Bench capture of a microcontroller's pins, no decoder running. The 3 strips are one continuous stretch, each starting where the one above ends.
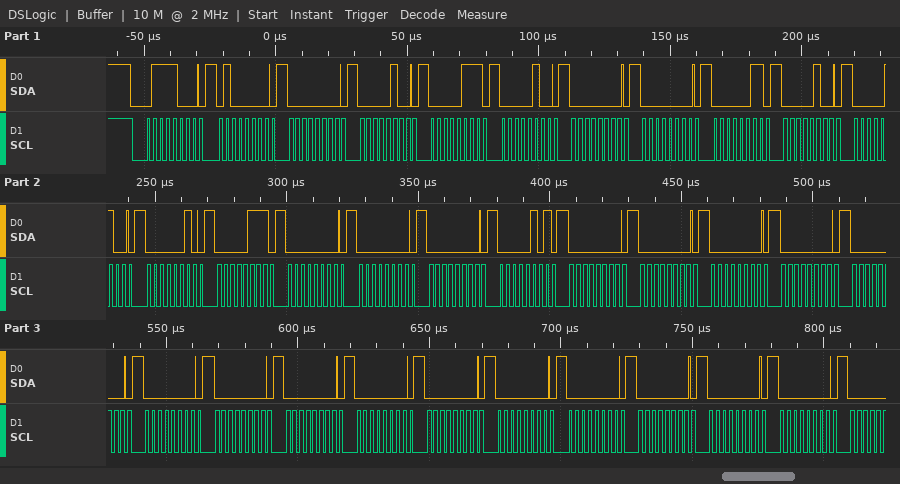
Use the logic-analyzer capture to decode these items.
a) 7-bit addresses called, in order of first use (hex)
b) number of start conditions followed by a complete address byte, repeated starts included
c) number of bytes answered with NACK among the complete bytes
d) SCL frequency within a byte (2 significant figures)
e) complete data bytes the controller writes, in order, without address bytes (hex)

0x3C
1
0
400 kHz
40 00 04 07 04 00 00 03 04 04 02 07 00 00 00 05 00 00 00 00 00 00 00 00 00 00 00 00 00 00 00
